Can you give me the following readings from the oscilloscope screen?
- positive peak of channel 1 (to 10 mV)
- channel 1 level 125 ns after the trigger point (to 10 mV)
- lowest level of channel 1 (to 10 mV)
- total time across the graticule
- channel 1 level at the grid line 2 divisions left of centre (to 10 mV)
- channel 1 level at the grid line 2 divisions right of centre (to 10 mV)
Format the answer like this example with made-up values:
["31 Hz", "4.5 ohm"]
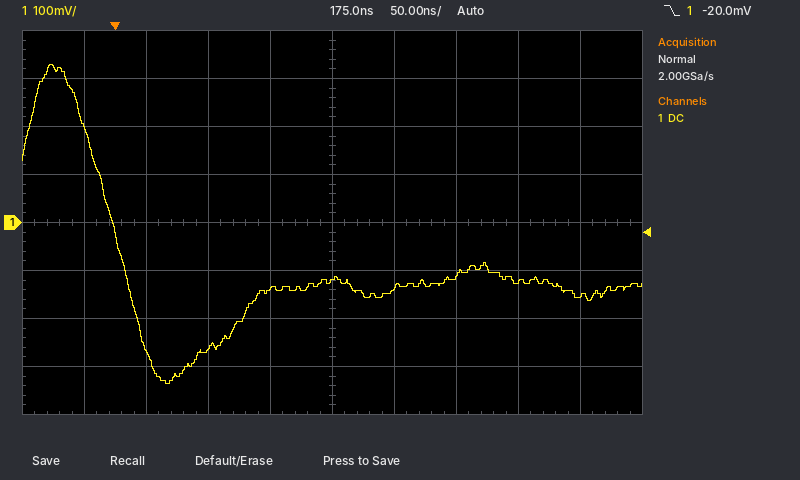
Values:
["330 mV", "-140 mV", "-340 mV", "500 ns", "-260 mV", "-110 mV"]
